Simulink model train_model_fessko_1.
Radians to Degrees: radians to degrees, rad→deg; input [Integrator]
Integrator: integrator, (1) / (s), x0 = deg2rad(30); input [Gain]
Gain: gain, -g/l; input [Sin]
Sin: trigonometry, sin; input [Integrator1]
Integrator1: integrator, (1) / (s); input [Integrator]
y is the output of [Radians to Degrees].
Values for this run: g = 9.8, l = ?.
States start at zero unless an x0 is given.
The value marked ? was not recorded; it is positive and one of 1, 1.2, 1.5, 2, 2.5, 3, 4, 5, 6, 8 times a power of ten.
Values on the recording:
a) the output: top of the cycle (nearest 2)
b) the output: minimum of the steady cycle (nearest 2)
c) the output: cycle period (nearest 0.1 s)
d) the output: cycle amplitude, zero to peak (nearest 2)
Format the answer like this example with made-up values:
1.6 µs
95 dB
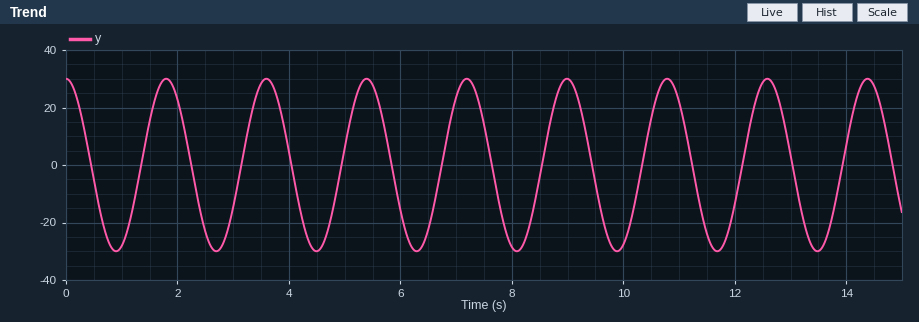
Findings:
30
-30
1.8 s
30
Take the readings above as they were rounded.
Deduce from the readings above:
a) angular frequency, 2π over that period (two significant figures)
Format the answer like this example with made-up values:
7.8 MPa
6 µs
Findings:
3.5 rad/s
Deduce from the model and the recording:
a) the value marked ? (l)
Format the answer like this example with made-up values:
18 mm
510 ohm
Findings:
0.8
